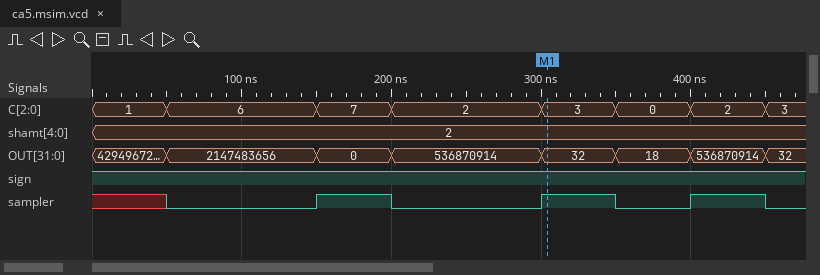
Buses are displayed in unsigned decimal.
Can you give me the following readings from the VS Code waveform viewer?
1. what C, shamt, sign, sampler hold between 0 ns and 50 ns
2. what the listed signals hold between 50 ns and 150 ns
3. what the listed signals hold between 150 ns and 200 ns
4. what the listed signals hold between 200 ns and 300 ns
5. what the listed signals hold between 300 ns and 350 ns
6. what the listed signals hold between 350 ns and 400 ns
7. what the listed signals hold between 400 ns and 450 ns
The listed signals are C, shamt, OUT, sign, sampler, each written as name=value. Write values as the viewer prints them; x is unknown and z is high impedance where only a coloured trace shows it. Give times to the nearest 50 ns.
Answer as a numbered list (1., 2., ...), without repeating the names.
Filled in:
1. C=1, shamt=2, sign=1, sampler=x
2. C=6, shamt=2, OUT=2147483656, sign=1, sampler=0
3. C=7, shamt=2, OUT=0, sign=1, sampler=1
4. C=2, shamt=2, OUT=536870914, sign=1, sampler=0
5. C=3, shamt=2, OUT=32, sign=1, sampler=1
6. C=0, shamt=2, OUT=18, sign=1, sampler=0
7. C=2, shamt=2, OUT=536870914, sign=1, sampler=1
